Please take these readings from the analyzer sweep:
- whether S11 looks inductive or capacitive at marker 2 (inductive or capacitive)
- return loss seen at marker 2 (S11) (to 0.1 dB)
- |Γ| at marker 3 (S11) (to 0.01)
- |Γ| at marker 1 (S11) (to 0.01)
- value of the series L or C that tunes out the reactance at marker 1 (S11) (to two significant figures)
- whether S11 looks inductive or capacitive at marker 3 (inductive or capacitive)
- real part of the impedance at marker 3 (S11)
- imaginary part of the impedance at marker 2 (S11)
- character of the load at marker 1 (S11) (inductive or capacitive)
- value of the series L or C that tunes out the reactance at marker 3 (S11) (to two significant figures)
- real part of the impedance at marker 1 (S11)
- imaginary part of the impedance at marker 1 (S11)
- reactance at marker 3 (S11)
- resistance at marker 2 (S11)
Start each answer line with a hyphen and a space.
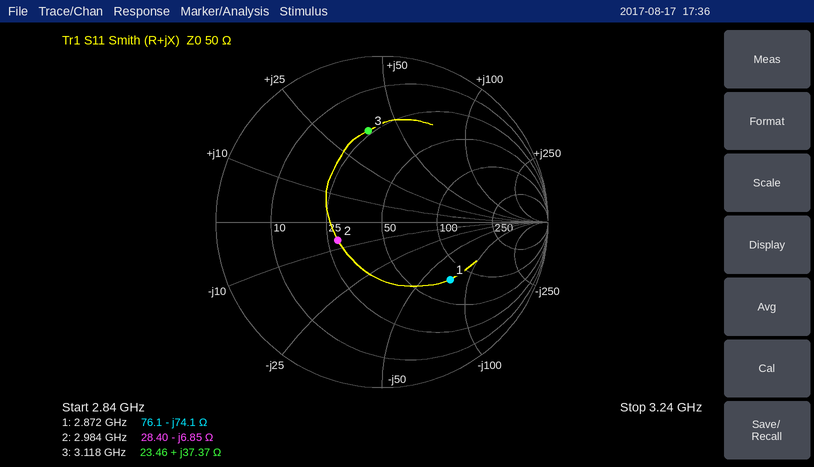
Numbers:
- capacitive
- 10.8 dB
- 0.56
- 0.54
- 4.1 nH
- inductive
- 23.46 Ω
- -6.85 Ω
- capacitive
- 1.4 pF
- 76.1 Ω
- -74.1 Ω
- +37.37 Ω
- 28.40 Ω
